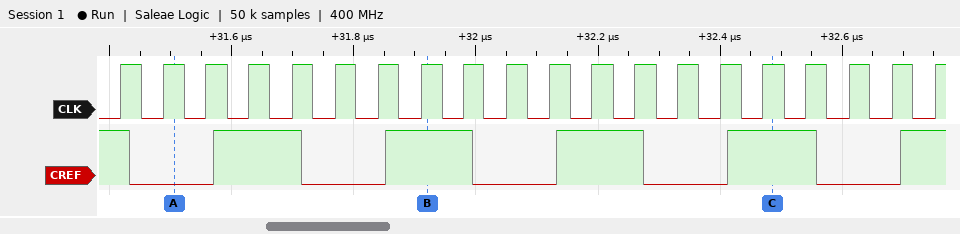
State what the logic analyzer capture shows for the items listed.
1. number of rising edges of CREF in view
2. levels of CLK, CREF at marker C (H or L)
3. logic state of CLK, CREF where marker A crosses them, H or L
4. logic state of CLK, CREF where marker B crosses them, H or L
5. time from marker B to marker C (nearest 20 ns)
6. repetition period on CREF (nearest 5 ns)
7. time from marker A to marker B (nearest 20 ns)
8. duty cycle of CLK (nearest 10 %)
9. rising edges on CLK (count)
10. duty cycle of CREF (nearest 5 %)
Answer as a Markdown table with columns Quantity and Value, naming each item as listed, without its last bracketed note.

| Quantity | Value |
|---|---|
| number of rising edges of CREF in view | 5 |
| levels of CLK, CREF at marker C | CLK=H, CREF=H |
| logic state of CLK, CREF where marker A crosses them, H or L | CLK=H, CREF=L |
| logic state of CLK, CREF where marker B crosses them, H or L | CLK=H, CREF=H |
| time from marker B to marker C | 560 ns |
| repetition period on CREF | 280 ns |
| time from marker A to marker B | 420 ns |
| duty cycle of CLK | 50 % |
| rising edges on CLK | 20 |
| duty cycle of CREF | 50 % |
